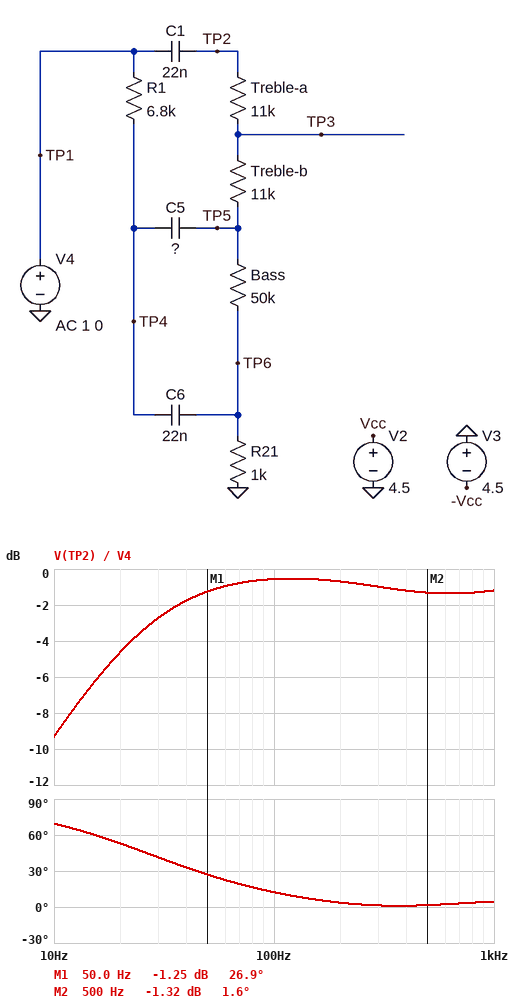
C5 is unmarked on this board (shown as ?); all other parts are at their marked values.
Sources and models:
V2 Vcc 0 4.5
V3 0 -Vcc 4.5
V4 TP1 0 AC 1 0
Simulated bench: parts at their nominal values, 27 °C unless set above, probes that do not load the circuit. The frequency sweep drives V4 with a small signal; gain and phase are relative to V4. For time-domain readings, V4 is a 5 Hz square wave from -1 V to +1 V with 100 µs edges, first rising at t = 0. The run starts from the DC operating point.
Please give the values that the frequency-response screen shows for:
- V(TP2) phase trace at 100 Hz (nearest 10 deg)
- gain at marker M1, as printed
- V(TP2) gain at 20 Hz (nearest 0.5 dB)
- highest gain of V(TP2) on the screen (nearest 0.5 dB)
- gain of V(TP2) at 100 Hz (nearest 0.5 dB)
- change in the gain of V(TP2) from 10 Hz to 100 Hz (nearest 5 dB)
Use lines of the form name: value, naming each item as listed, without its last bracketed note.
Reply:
V(TP2) phase trace at 100 Hz: 10 deg
gain at marker M1, as printed: -1.25 dB
V(TP2) gain at 20 Hz: -4.5 dB
highest gain of V(TP2) on the screen: -0.5 dB
gain of V(TP2) at 100 Hz: -0.5 dB
change in the gain of V(TP2) from 10 Hz to 100 Hz: 10 dB
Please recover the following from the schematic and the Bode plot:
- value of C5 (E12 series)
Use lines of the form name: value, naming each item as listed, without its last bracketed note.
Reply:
value of C5: 82 nF
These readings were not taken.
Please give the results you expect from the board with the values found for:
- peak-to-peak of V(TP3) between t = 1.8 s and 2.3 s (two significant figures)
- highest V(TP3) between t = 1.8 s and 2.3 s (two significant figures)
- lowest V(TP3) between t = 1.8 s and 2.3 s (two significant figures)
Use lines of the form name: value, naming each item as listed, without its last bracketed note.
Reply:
peak-to-peak of V(TP3) between t = 1.8 s and 2.3 s: 3.3 V
highest V(TP3) between t = 1.8 s and 2.3 s: 1.7 V
lowest V(TP3) between t = 1.8 s and 2.3 s: -1.7 V
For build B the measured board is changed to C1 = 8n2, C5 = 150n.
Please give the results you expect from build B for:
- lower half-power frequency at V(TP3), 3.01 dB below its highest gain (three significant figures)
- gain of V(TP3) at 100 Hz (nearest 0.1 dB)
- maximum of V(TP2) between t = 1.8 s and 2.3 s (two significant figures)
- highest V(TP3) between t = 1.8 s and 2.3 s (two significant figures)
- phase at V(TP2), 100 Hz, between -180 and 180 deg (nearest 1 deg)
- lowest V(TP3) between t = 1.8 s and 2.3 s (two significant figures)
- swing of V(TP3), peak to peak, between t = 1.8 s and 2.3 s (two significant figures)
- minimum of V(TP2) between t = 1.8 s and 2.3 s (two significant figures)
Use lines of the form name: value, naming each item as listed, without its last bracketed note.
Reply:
lower half-power frequency at V(TP3), 3.01 dB below its highest gain: 16.8 Hz
gain of V(TP3) at 100 Hz: -1.1 dB
maximum of V(TP2) between t = 1.8 s and 2.3 s: 1.7 V
highest V(TP3) between t = 1.8 s and 2.3 s: 1.6 V
phase at V(TP2), 100 Hz, between -180 and 180 deg: 7 deg
lowest V(TP3) between t = 1.8 s and 2.3 s: -1.6 V
swing of V(TP3), peak to peak, between t = 1.8 s and 2.3 s: 3.3 V
minimum of V(TP2) between t = 1.8 s and 2.3 s: -1.7 V
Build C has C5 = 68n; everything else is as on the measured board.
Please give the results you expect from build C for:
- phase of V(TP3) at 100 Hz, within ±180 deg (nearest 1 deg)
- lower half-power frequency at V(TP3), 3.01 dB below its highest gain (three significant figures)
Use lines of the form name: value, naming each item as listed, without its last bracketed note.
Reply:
phase of V(TP3) at 100 Hz, within ±180 deg: 14 deg
lower half-power frequency at V(TP3), 3.01 dB below its highest gain: 28.8 Hz
